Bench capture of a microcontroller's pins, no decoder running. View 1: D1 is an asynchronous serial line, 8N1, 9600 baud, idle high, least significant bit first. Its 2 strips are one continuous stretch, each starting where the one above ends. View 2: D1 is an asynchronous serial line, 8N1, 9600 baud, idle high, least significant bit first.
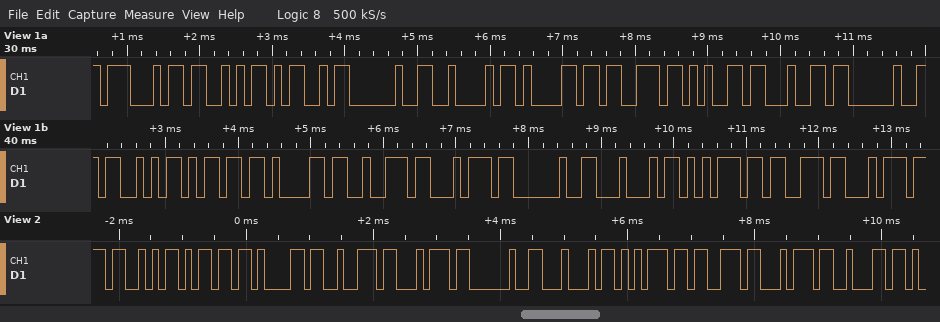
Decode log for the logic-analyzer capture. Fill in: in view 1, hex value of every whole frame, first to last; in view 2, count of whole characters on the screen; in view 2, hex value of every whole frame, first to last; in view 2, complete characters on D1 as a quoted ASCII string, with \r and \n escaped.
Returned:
47 53 4D 20 42 61 73 65 64 20 53 6D 61 72 74 20 44 75 73 74
11
0x53 0x6D 0x61 0x72 0x74 0x20 0x44 0x75 0x73 0x74 0x62
"Smart Dustb"
